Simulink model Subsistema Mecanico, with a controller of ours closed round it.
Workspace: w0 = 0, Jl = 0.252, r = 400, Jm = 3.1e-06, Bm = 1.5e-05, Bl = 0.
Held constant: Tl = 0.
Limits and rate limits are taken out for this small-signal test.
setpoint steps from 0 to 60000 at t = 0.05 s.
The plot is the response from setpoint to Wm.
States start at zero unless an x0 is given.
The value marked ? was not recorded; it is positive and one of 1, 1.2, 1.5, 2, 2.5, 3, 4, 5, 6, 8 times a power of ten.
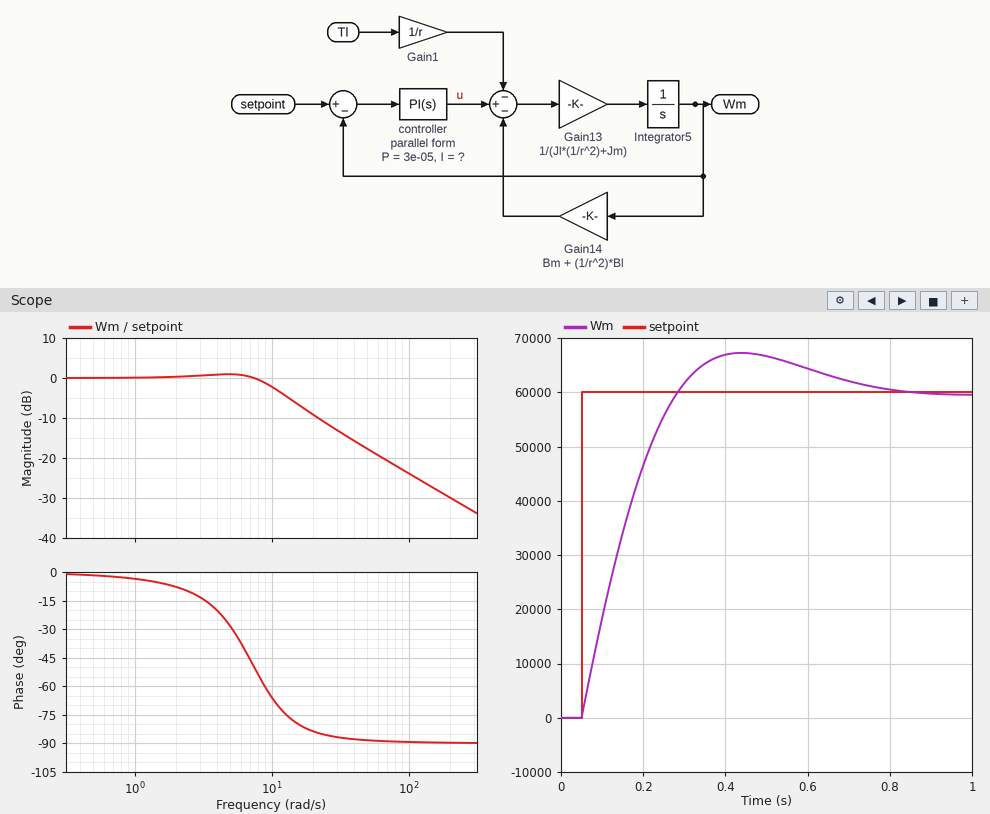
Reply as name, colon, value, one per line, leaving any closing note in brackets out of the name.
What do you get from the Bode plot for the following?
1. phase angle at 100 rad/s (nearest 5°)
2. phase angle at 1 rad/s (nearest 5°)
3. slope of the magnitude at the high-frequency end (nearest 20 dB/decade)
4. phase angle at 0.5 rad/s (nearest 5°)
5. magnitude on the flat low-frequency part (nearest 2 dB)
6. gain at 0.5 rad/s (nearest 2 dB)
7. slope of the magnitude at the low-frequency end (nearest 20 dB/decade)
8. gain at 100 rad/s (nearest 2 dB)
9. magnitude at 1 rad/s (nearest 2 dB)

phase angle at 100 rad/s: -90°
phase angle at 1 rad/s: -5°
slope of the magnitude at the high-frequency end: -20 dB/decade
phase angle at 0.5 rad/s: 0°
magnitude on the flat low-frequency part: 0 dB
gain at 0.5 rad/s: 0 dB
slope of the magnitude at the low-frequency end: 0 dB/decade
gain at 100 rad/s: -24 dB
magnitude at 1 rad/s: 0 dB
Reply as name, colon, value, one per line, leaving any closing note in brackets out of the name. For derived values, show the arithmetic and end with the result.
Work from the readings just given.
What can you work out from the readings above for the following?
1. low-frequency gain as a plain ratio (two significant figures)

low-frequency gain as a plain ratio: 10^(0 / 20) = 1.0
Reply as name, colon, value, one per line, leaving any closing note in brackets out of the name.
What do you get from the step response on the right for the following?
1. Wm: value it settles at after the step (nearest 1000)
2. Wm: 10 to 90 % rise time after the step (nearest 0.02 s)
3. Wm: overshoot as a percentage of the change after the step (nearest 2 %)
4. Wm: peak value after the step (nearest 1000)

Wm: value it settles at after the step: 60000
Wm: 10 to 90 % rise time after the step: 0.18 s
Wm: overshoot as a percentage of the change after the step: 12 %
Wm: peak value after the step: 67000
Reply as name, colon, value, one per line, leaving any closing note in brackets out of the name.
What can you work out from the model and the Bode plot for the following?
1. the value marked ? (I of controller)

the value marked ?: 0.00025
